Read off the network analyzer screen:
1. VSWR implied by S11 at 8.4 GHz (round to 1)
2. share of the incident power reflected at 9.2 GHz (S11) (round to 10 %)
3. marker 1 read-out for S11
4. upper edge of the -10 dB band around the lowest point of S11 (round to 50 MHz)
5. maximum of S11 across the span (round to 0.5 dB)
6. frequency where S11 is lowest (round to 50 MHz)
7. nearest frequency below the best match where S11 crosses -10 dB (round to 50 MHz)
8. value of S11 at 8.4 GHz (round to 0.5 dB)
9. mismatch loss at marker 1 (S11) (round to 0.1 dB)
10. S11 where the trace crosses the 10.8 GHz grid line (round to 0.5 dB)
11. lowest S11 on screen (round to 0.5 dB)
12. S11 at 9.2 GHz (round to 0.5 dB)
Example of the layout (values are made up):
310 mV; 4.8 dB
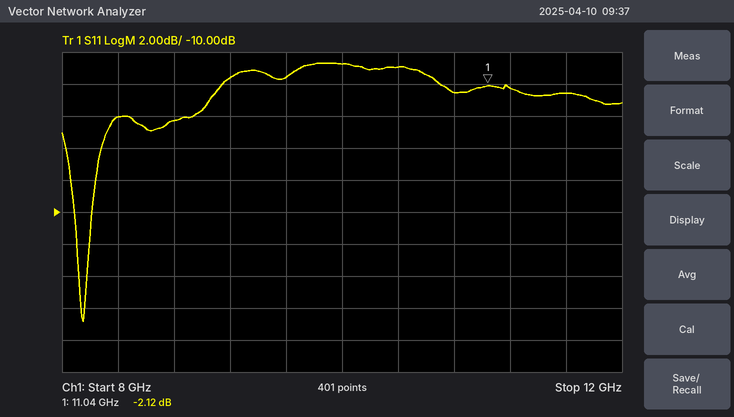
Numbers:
4; 70 %; -2.12 dB; 8.20 GHz; -0.5 dB; 8.15 GHz; 8.10 GHz; -4.0 dB; 4.1 dB; -2.5 dB; -17.0 dB; -1.5 dB
